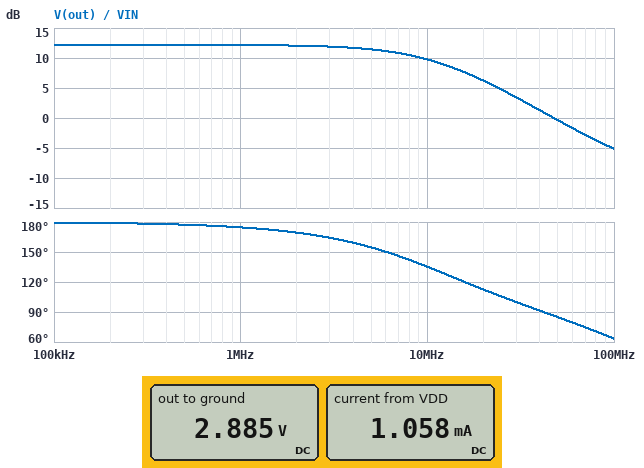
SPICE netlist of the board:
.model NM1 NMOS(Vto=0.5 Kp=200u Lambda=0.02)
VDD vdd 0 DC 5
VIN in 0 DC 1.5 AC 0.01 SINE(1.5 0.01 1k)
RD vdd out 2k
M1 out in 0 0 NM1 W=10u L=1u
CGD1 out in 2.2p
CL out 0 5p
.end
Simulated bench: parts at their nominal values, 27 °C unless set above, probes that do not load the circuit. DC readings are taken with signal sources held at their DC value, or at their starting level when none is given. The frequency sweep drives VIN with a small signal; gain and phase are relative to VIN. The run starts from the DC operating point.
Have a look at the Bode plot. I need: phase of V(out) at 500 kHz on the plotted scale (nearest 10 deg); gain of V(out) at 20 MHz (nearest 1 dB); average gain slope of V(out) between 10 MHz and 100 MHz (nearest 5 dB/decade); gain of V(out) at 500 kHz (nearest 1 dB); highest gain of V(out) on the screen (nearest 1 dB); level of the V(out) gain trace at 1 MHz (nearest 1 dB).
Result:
180 deg
6 dB
-15 dB/decade
12 dB
12 dB
12 dB
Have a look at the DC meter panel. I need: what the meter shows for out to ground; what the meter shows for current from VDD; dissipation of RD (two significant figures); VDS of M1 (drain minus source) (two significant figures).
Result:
2.885 V
1.058 mA
2.2 mW
2.9 V
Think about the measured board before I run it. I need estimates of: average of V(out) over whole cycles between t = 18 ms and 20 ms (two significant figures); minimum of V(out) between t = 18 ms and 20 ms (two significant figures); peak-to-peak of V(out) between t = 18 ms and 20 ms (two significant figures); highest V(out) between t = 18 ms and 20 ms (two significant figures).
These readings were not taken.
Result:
2.9 V
2.8 V
81 mV
2.9 V
